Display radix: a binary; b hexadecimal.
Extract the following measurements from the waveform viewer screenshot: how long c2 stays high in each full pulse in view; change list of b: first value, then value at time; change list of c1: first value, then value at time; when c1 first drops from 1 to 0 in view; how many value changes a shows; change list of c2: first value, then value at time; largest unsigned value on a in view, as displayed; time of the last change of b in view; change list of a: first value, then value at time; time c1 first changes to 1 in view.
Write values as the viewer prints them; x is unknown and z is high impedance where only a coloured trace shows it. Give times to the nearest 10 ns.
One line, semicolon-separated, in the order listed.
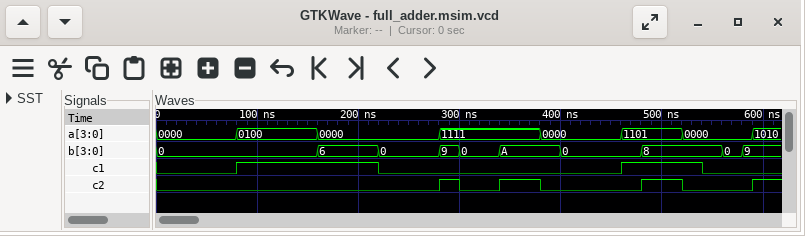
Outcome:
20 ns, 40 ns, 40 ns; 0, 6 at 160 ns, 0 at 220 ns, 9 at 280 ns, 0 at 300 ns, A at 340 ns, 0 at 400 ns, 8 at 480 ns, 0 at 560 ns, 9 at 580 ns; 0, 1 at 80 ns, 0 at 220 ns, 1 at 460 ns, 0 at 540 ns; 220 ns; 7; 0, 1 at 280 ns, 0 at 300 ns, 1 at 340 ns, 0 at 380 ns, 1 at 480 ns, 0 at 520 ns, 1 at 590 ns; 1111; 580 ns; 0000, 0100 at 80 ns, 0000 at 160 ns, 1111 at 280 ns, 0000 at 380 ns, 1101 at 460 ns, 0000 at 520 ns, 1010 at 590 ns; 80 ns
